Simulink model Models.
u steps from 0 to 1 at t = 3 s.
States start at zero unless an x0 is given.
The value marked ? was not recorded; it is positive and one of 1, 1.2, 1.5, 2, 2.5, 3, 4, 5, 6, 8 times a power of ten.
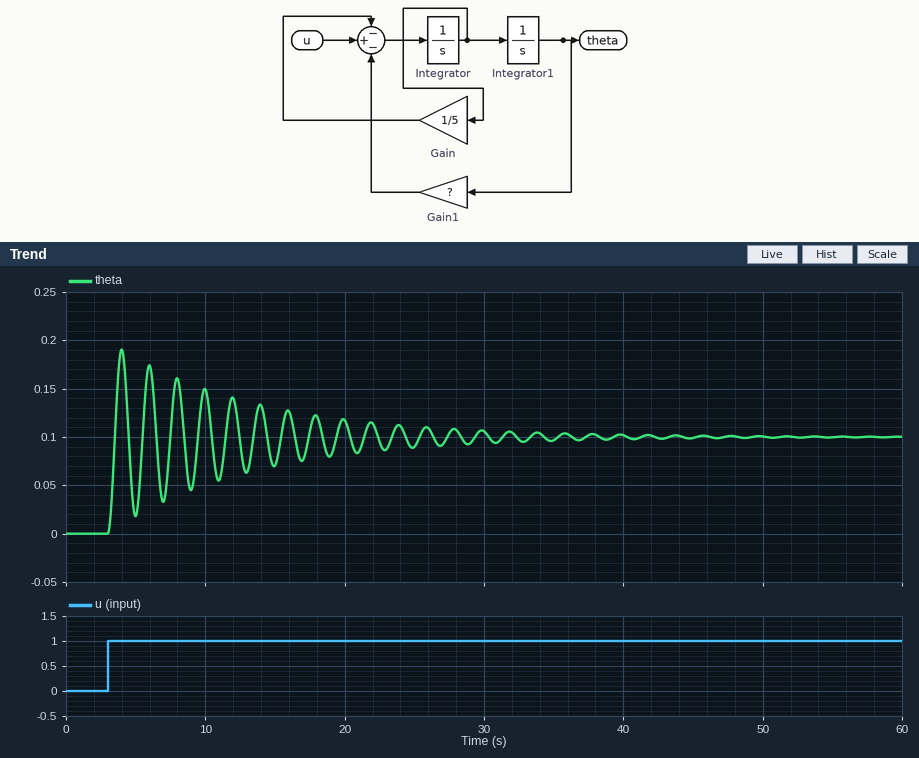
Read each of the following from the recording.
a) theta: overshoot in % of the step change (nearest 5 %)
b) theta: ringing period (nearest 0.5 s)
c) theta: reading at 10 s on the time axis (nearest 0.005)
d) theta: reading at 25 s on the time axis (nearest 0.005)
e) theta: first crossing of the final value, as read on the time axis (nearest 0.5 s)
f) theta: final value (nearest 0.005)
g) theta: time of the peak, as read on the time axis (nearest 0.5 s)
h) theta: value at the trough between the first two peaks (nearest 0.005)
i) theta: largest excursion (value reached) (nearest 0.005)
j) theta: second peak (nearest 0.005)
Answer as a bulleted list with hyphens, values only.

- 90 %
- 2.0 s
- 0.150
- 0.090
- 3.5 s
- 0.100
- 4.0 s
- 0.020
- 0.190
- 0.175
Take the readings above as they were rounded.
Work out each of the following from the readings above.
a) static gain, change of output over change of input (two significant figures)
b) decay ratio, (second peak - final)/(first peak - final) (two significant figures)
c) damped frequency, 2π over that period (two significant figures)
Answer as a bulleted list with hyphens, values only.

- 0.10
- 0.83
- 3.1 rad/s
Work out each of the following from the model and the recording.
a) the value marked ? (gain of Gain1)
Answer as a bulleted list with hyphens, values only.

- 10
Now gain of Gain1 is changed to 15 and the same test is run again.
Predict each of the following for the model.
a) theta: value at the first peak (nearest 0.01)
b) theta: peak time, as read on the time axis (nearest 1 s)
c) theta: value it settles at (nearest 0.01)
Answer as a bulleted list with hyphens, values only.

- 0.13
- 4 s
- 0.07
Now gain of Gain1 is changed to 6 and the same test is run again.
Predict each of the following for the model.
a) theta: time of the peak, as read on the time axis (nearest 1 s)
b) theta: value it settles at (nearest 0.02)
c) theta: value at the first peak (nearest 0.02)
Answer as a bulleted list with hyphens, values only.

- 4 s
- 0.16
- 0.32
